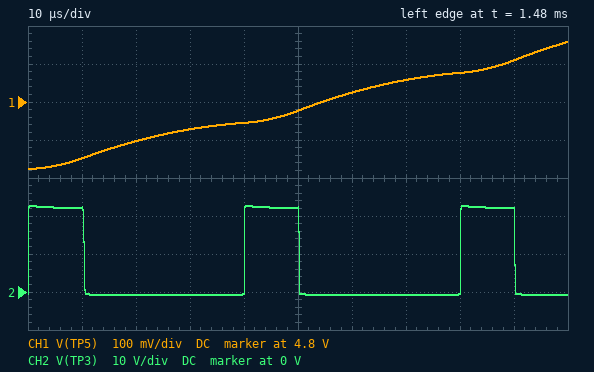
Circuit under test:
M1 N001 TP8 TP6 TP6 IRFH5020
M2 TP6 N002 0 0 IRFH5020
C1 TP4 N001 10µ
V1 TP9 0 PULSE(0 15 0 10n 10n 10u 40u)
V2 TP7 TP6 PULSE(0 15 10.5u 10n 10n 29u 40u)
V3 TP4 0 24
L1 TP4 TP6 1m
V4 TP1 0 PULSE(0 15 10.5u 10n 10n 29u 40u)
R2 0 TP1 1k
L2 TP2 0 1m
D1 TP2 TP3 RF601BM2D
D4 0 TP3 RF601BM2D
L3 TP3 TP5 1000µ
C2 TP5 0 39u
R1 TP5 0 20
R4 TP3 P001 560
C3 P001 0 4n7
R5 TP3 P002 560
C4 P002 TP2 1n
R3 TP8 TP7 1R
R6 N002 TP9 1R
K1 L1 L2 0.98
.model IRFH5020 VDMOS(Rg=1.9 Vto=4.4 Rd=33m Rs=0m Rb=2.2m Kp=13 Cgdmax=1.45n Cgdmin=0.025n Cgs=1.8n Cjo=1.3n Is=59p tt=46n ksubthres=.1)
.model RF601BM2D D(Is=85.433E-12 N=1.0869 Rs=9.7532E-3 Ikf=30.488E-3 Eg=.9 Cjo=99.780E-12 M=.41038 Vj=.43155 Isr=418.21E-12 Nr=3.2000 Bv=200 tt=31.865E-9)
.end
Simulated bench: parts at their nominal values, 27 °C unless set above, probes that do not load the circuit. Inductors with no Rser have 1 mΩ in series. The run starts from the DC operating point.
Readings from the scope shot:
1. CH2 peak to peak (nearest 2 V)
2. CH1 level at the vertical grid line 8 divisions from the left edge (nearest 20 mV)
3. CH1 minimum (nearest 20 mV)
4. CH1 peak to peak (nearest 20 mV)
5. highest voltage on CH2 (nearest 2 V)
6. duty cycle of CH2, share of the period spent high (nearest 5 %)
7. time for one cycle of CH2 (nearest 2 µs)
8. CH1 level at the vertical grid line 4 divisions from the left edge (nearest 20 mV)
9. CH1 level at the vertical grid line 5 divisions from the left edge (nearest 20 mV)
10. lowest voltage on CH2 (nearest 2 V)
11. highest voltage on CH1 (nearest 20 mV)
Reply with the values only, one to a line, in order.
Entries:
24 V
4.88 V
4.62 V
340 mV
22 V
25 %
40 µs
4.74 V
4.78 V
0 V
4.96 V
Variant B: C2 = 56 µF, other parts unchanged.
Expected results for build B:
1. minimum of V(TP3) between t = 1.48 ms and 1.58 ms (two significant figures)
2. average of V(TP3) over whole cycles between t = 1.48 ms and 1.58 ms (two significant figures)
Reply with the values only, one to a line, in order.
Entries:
-690 mV
5.5 V
